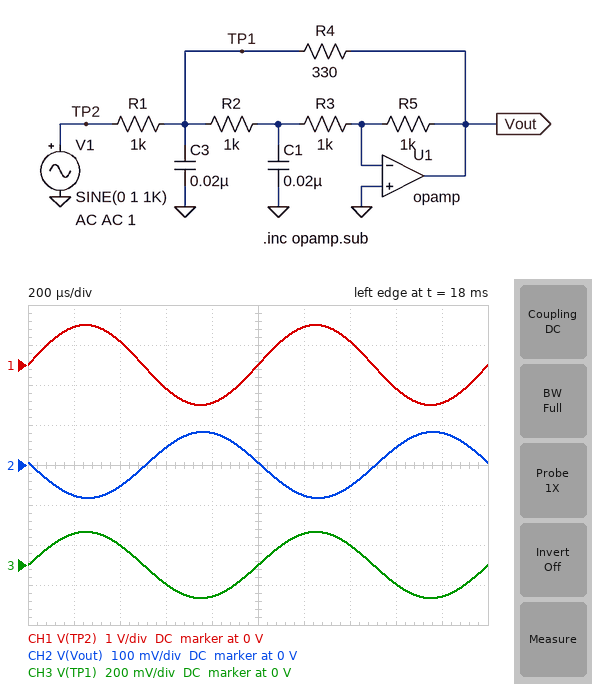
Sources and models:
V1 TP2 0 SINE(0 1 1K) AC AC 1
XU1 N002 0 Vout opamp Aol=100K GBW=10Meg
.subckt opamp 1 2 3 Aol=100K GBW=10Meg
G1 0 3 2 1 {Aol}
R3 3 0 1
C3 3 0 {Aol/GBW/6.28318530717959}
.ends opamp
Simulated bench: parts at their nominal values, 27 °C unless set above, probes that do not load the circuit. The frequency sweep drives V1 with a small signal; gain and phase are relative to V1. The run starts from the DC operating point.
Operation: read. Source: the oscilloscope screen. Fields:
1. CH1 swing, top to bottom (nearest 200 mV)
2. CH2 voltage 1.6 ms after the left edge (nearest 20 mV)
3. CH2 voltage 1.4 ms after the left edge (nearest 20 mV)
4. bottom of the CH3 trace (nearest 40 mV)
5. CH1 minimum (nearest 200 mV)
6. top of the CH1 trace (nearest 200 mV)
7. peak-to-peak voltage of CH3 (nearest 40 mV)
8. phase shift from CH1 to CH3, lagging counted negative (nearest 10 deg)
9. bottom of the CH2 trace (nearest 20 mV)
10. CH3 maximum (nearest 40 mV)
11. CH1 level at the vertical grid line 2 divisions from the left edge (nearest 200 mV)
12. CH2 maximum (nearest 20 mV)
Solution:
2.0 V
40 mV
-60 mV
-160 mV
-1.0 V
1.0 V
320 mV
0 deg
-80 mV
160 mV
600 mV
80 mV
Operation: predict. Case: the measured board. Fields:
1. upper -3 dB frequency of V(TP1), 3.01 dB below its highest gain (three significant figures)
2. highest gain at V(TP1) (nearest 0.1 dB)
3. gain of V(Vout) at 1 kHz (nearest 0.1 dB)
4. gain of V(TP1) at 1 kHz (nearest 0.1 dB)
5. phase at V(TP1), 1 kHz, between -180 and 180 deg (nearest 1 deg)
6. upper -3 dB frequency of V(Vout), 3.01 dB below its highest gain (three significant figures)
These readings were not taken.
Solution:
52.3 kHz
-15.2 dB
-21.7 dB
-15.6 dB
-1 deg
17.6 kHz
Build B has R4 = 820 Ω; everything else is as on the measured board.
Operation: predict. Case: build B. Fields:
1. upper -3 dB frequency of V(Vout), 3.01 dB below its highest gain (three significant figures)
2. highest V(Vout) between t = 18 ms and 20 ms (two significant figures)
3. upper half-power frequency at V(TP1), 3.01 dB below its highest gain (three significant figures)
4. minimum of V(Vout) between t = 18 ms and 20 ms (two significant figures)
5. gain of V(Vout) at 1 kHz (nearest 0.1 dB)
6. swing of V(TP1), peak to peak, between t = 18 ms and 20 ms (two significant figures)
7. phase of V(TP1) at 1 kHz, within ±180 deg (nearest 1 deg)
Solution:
13.0 kHz
150 mV
27.5 kHz
-150 mV
-16.5 dB
600 mV
-2 deg
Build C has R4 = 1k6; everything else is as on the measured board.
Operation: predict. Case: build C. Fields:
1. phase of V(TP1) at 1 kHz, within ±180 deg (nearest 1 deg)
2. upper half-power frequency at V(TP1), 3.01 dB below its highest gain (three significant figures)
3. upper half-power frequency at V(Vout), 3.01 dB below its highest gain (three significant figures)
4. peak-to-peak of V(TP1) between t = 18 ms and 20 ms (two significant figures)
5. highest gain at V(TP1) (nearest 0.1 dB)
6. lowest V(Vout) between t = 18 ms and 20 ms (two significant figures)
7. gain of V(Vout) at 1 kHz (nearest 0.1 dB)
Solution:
-3 deg
17.8 kHz
10.6 kHz
820 mV
-7.7 dB
-200 mV
-13.8 dB
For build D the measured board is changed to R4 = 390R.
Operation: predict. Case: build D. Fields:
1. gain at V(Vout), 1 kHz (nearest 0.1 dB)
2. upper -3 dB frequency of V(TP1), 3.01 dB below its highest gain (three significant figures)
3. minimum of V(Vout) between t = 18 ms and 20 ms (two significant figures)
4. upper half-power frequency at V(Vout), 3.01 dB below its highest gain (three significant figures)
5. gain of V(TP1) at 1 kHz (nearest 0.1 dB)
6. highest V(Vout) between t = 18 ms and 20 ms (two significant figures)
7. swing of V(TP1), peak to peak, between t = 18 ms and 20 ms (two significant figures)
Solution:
-20.6 dB
47.1 kHz
-93 mV
16.7 kHz
-14.6 dB
93 mV
370 mV
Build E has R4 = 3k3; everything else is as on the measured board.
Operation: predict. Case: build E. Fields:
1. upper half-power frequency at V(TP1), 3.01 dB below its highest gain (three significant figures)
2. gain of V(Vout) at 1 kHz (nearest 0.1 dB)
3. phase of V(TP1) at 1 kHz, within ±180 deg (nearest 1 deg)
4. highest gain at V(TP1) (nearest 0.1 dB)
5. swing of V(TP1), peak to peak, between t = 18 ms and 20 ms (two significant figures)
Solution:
13.0 kHz
-11.9 dB
-4 deg
-5.8 dB
1.0 V
